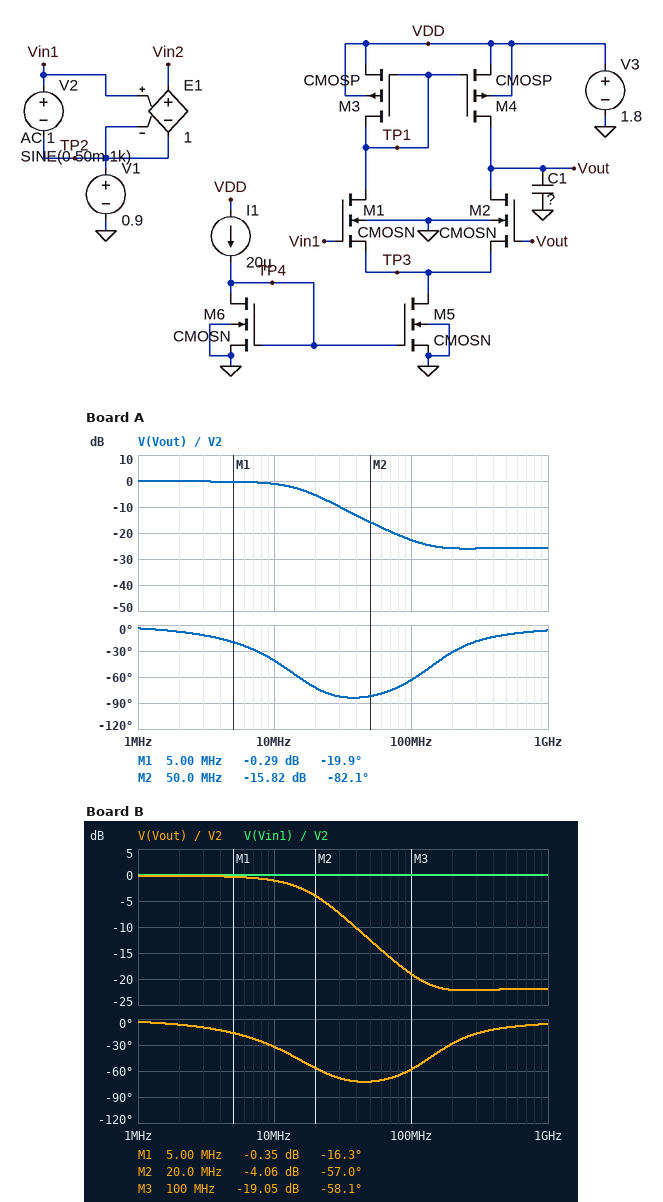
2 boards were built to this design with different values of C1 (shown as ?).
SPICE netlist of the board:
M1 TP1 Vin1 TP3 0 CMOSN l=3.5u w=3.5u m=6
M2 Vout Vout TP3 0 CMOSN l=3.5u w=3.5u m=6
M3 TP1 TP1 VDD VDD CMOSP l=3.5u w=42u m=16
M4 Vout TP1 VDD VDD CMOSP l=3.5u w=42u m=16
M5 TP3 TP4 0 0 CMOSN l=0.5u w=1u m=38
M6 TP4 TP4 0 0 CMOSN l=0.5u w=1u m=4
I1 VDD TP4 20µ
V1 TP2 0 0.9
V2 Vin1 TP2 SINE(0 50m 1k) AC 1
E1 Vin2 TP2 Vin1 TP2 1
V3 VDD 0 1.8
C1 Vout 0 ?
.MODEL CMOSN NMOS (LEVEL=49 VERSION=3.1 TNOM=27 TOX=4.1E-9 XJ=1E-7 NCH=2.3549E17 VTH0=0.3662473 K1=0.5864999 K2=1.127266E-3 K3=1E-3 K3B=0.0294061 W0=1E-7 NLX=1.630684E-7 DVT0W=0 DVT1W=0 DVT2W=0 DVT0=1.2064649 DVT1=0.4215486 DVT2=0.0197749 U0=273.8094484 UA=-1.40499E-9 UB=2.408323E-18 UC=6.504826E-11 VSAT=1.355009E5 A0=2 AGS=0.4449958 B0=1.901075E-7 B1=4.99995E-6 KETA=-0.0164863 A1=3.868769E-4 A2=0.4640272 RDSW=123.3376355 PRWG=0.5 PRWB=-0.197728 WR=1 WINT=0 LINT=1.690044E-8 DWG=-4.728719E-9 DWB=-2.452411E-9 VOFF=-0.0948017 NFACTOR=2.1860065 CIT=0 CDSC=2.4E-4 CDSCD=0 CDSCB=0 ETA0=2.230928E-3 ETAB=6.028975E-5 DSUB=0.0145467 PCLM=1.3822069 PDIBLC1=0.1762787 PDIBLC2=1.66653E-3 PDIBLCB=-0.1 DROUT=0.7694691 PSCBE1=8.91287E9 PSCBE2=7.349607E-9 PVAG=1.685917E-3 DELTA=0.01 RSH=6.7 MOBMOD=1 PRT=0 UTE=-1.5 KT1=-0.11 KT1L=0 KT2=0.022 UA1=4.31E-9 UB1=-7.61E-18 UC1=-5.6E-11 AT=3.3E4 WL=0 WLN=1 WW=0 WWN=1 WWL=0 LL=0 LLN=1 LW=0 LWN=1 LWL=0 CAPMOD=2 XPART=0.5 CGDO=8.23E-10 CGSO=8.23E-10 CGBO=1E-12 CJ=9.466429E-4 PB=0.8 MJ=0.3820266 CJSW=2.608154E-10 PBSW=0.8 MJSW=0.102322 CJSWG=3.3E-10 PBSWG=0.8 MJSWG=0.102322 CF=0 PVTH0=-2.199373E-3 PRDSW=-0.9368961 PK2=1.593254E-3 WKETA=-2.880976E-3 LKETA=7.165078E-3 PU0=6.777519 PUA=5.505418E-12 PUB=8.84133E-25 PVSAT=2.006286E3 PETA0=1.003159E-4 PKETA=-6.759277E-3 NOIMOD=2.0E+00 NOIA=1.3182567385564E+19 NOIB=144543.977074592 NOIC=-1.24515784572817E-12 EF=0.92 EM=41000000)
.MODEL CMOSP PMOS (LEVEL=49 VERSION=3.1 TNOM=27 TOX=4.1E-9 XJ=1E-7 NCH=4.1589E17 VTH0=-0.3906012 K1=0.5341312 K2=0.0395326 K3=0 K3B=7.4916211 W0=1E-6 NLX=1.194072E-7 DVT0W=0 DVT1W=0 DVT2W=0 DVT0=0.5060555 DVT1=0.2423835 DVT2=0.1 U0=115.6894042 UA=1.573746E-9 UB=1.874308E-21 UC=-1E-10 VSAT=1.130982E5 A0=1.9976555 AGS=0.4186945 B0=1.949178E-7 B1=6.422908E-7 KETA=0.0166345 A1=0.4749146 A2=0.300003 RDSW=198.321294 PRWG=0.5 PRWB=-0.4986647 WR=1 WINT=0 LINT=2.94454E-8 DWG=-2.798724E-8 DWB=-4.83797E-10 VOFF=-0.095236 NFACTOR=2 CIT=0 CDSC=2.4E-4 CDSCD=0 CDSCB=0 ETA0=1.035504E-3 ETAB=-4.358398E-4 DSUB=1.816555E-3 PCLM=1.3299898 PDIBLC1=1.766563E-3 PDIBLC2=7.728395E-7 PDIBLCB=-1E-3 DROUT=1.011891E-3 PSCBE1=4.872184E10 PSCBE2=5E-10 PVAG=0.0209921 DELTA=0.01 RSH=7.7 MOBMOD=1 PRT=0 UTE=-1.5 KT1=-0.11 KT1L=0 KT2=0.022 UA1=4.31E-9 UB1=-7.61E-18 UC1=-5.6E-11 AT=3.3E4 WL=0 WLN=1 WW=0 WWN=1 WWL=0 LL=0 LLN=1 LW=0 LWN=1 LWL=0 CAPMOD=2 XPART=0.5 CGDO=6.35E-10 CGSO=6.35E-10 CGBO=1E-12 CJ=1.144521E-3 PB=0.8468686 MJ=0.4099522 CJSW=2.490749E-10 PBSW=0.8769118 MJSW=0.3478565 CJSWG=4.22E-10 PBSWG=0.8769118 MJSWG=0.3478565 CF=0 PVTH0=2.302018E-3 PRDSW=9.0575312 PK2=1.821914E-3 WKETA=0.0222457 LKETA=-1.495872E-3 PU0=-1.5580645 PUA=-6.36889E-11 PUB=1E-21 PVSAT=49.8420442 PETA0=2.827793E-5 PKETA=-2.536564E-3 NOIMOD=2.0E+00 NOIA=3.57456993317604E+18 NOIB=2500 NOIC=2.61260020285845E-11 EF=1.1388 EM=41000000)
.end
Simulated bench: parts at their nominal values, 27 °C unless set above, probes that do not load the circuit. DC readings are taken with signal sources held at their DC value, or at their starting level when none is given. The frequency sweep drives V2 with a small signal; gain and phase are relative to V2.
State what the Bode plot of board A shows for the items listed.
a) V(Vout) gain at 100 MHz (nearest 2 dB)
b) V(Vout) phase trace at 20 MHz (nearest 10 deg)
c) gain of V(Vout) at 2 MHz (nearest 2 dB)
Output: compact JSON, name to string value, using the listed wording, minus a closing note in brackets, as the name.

{"V(Vout) gain at 100 MHz": "-22 dB", "V(Vout) phase trace at 20 MHz": "-70 deg", "gain of V(Vout) at 2 MHz": "0 dB"}
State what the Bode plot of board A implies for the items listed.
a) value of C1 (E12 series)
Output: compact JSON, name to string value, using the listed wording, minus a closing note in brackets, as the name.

{"value of C1": "1.5 pF"}
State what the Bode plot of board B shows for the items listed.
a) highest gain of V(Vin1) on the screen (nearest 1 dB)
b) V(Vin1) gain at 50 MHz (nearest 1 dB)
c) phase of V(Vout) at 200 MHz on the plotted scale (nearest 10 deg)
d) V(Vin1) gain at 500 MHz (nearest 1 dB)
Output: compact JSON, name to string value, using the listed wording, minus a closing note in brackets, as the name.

{"highest gain of V(Vin1) on the screen": "0 dB", "V(Vin1) gain at 50 MHz": "0 dB", "phase of V(Vout) at 200 MHz on the plotted scale": "-30 deg", "V(Vin1) gain at 500 MHz": "0 dB"}
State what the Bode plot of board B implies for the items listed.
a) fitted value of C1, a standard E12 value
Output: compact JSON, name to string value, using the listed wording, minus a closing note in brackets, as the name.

{"fitted value of C1, a standard E12 value": "680 fF"}
